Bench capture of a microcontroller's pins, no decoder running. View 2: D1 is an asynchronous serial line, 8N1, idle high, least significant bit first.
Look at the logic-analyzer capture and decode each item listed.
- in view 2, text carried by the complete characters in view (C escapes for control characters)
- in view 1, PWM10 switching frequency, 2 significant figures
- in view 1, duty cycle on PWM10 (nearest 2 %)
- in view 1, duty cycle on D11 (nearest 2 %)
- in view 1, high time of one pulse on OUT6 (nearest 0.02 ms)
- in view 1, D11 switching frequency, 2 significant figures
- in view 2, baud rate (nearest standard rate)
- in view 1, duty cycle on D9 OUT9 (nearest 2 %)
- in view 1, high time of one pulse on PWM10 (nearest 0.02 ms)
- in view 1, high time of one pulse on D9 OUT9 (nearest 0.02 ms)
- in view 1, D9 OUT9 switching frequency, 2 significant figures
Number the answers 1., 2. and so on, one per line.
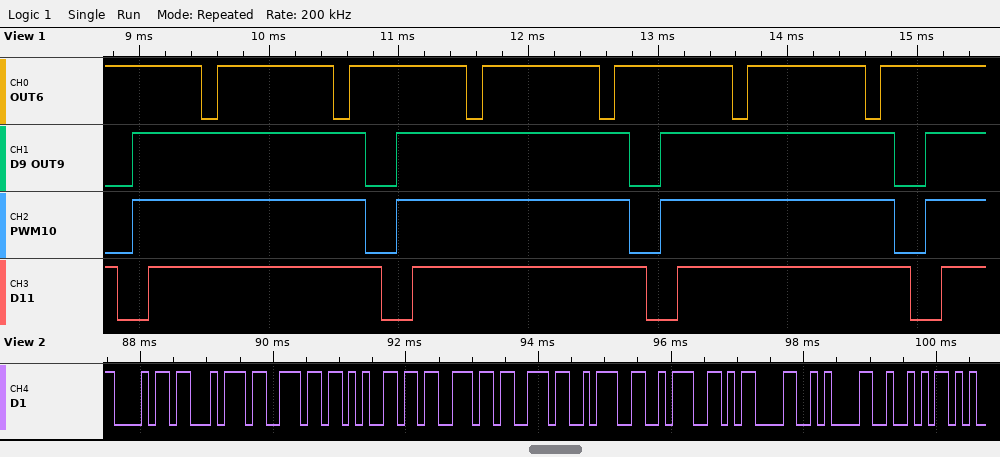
1. "htness::\r\nR"
2. 490 Hz
3. 88 %
4. 88 %
5. 0.90 ms
6. 490 Hz
7. 9600 baud
8. 88 %
9. 1.80 ms
10. 1.80 ms
11. 490 Hz
